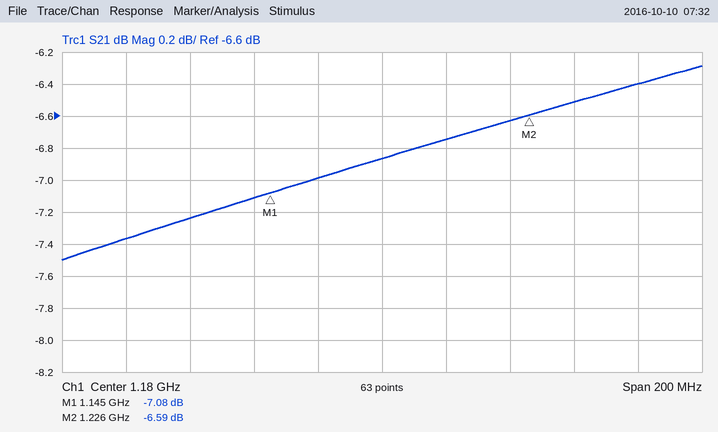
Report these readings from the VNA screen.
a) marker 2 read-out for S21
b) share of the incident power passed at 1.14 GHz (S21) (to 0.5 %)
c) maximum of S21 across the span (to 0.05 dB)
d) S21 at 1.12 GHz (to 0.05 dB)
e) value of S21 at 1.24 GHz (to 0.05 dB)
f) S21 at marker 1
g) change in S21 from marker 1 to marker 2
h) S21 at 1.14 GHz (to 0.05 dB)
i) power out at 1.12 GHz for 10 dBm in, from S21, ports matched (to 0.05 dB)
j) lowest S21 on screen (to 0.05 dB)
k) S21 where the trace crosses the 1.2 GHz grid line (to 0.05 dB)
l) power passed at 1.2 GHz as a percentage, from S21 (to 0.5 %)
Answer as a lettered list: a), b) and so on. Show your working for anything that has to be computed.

a) -6.59 dB
b) 10^(-7.1/10) ≈ 19.5 %
c) -6.30 dB
d) -7.25 dB
e) -6.50 dB
f) -7.08 dB
g) -6.59 − (-7.08) = 0.49 dB
h) -7.10 dB
i) 10 dBm + (-7.25 dB) = 2.75 dBm
j) -7.50 dB
k) -6.75 dB
l) 10^(-6.75/10) ≈ 21.1 %, so 21.0 % to the nearest 0.5 %
